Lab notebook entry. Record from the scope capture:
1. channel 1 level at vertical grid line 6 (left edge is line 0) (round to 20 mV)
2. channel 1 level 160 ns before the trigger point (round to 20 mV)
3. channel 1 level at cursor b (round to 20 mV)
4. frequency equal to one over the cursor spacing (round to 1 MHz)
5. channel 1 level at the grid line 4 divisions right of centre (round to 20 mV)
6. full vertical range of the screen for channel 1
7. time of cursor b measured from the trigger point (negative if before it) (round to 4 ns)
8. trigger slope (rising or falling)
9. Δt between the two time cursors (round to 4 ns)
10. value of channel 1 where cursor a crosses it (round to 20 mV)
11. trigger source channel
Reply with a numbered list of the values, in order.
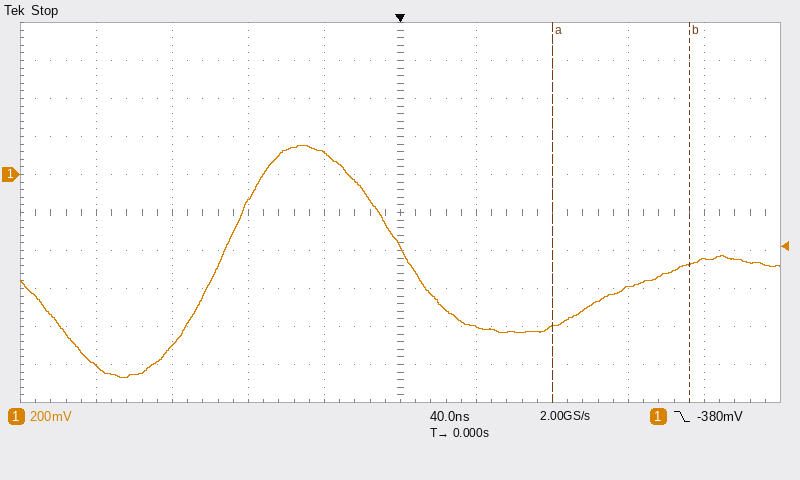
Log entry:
1. -800 mV
2. -1.00 V
3. -480 mV
4. 14 MHz
5. -440 mV
6. 2 V
7. +152 ns
8. falling
9. 72 ns
10. -800 mV
11. channel 1
